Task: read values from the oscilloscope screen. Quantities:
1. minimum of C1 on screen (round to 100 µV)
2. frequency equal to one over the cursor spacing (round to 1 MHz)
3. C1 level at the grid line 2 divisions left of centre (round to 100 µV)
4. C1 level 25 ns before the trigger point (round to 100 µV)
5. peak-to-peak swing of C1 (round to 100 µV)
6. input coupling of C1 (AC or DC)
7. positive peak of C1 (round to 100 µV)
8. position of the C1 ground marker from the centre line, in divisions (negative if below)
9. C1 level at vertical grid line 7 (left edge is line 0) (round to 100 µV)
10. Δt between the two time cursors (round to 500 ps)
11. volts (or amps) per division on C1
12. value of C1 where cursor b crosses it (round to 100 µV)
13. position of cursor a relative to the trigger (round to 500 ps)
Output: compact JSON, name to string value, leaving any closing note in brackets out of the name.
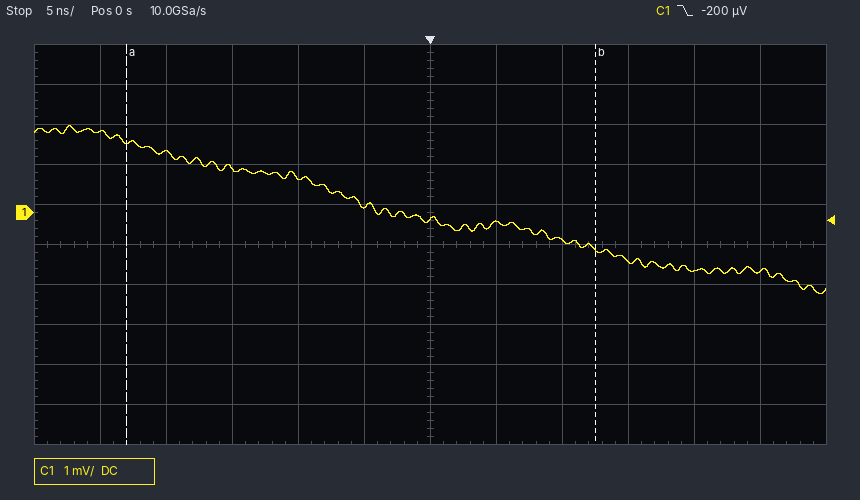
{"minimum of C1 on screen": "-2.0 mV", "frequency equal to one over the cursor spacing": "28 MHz", "C1 level at the grid line 2 divisions left of centre": "900 µV", "C1 level 25 ns before the trigger point": "2.0 mV", "peak-to-peak swing of C1": "4.2 mV", "input coupling of C1": "DC", "positive peak of C1": "2.2 mV", "position of the C1 ground marker from the centre line, in divisions": "+0.8 div", "C1 level at vertical grid line 7 (left edge is line 0)": "-200 µV", "Δt between the two time cursors": "35.5 ns", "volts (or amps) per division on C1": "1 mV", "value of C1 where cursor b crosses it": "-900 µV", "position of cursor a relative to the trigger": "-23.0 ns"}
